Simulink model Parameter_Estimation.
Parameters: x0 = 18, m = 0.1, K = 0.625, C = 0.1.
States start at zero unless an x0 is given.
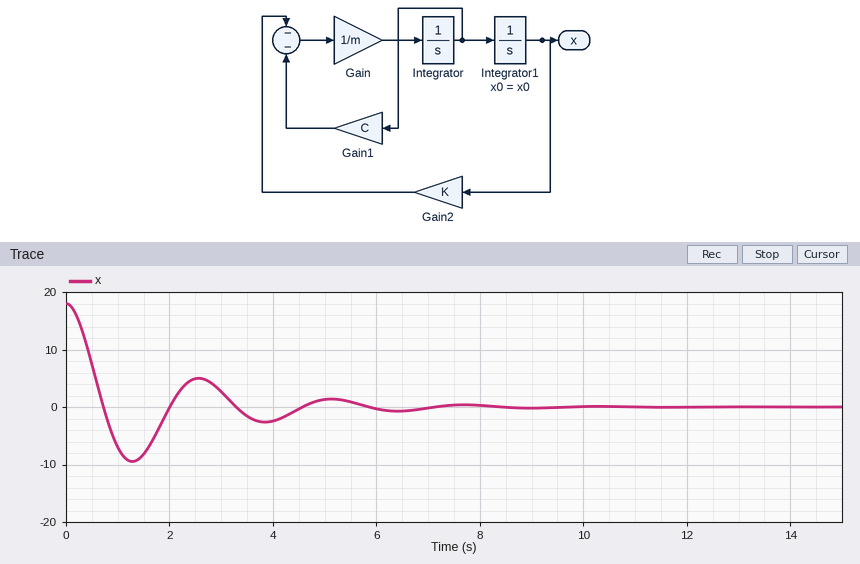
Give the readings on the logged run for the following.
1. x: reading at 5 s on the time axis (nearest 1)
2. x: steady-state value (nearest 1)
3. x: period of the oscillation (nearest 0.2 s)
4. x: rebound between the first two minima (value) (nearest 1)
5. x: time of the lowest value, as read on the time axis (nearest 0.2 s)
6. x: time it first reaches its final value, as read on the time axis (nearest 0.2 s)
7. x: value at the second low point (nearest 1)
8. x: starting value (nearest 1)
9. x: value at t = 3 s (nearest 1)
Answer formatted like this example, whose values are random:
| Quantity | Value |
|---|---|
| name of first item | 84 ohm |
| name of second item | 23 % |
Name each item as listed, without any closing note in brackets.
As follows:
| Quantity | Value |
|---|---|
| x: reading at 5 s on the time axis | 1 |
| x: steady-state value | 0 |
| x: period of the oscillation | 2.6 s |
| x: rebound between the first two minima (value) | 5 |
| x: time of the lowest value, as read on the time axis | 1.2 s |
| x: time it first reaches its final value, as read on the time axis | 0.8 s |
| x: value at the second low point | -3 |
| x: starting value | 18 |
| x: value at t = 3 s | 3 |
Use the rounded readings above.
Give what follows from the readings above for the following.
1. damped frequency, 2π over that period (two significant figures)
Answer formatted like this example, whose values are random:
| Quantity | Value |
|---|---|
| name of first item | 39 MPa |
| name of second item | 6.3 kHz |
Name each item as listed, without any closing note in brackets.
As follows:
| Quantity | Value |
|---|---|
| damped frequency, 2π over that period | 2.4 rad/s |
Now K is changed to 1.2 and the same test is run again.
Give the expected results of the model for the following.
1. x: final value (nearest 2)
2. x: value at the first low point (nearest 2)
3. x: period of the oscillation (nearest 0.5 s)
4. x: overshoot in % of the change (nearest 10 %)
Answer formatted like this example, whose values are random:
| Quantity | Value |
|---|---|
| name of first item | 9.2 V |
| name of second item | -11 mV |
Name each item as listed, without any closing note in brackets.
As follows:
| Quantity | Value |
|---|---|
| x: final value | 0 |
| x: value at the first low point | -12 |
| x: period of the oscillation | 2.0 s |
| x: overshoot in % of the change | 60 % |
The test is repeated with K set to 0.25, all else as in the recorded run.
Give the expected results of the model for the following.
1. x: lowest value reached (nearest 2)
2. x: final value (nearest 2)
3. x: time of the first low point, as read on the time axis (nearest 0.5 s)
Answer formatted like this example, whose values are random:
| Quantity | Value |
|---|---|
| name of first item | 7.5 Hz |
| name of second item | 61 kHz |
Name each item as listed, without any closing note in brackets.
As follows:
| Quantity | Value |
|---|---|
| x: lowest value reached | -6 |
| x: final value | 0 |
| x: time of the first low point, as read on the time axis | 2.0 s |
